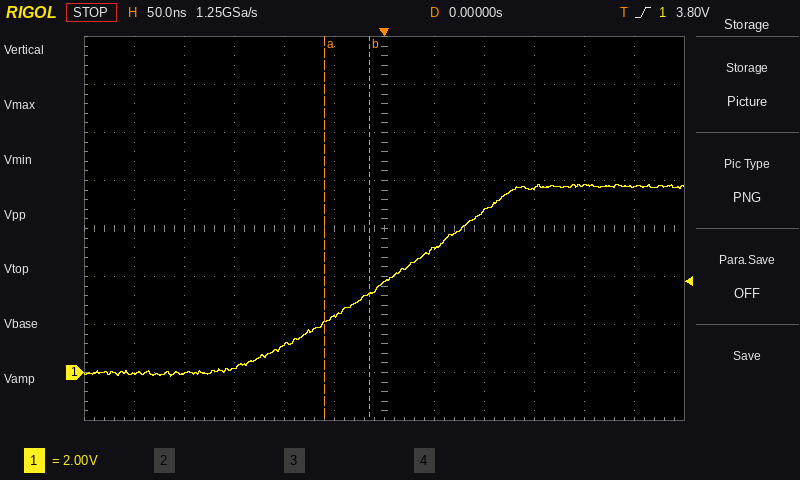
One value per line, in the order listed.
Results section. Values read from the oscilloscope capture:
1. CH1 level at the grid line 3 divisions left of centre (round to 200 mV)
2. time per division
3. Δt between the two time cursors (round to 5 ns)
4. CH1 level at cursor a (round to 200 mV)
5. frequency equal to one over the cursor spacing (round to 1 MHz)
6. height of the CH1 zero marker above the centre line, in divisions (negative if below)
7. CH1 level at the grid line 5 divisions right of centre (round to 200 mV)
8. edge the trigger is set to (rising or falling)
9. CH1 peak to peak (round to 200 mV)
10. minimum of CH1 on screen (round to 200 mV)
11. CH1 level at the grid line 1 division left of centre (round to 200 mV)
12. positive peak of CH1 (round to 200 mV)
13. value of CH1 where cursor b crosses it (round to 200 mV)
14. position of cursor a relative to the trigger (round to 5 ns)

200 mV
50 ns
45 ns
2.0 V
22 MHz
-3.0 div
7.8 V
rising
8.0 V
-200 mV
2.4 V
7.8 V
3.2 V
-60 ns
